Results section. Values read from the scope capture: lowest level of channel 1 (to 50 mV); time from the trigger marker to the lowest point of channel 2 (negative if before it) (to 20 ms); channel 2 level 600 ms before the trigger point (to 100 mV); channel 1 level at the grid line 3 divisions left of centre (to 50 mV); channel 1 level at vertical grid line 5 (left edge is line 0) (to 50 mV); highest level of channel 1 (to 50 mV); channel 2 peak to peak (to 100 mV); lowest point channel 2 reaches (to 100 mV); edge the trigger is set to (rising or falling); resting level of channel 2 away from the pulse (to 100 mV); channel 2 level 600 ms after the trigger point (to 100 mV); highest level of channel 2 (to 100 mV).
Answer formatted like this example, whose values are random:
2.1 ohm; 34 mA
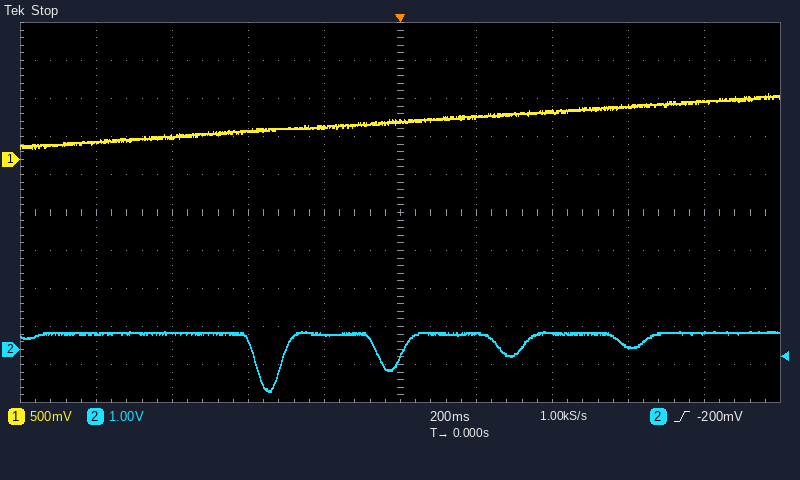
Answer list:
150 mV; -340 ms; 400 mV; 300 mV; 500 mV; 850 mV; 1.6 V; -1.1 V; rising; 400 mV; 100 mV; 500 mV
